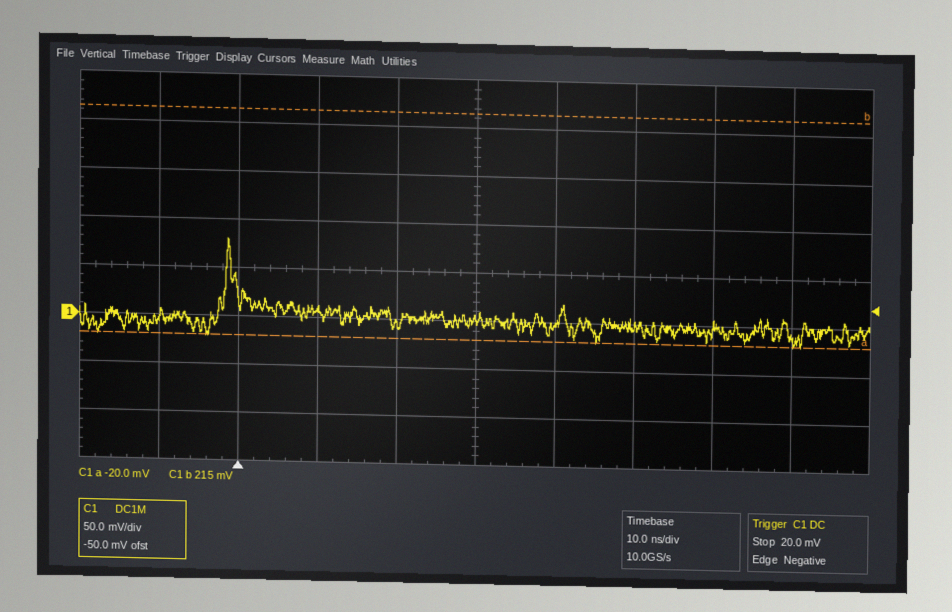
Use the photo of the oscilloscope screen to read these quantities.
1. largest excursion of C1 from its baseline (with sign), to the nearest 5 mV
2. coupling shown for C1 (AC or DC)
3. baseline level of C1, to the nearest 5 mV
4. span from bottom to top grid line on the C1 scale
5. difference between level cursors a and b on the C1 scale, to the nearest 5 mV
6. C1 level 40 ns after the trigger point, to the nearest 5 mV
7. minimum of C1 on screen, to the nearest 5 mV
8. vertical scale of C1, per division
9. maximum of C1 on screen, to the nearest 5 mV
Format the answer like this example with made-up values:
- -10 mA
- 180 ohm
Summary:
- +80 mV
- DC
- 0 mV
- 400 mV
- 235 mV
- 0 mV
- -20 mV
- 50 mV
- 80 mV
